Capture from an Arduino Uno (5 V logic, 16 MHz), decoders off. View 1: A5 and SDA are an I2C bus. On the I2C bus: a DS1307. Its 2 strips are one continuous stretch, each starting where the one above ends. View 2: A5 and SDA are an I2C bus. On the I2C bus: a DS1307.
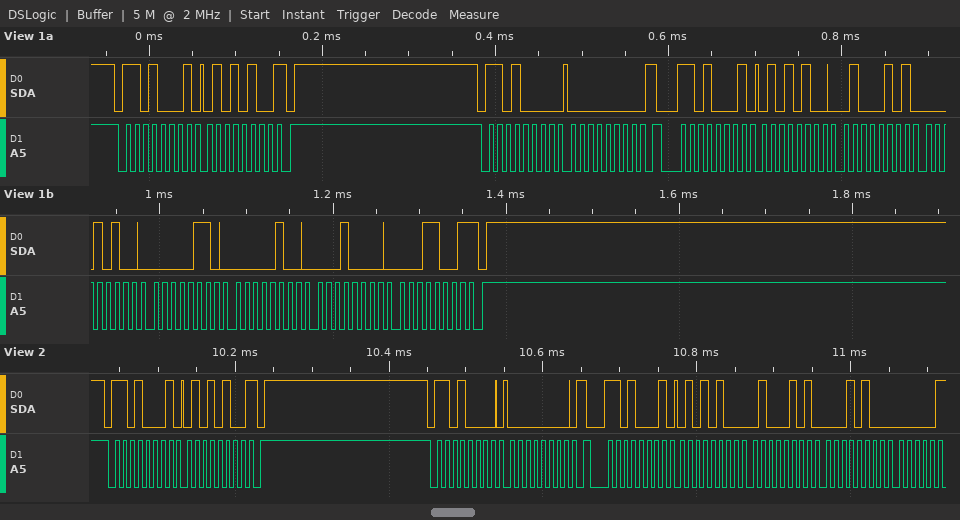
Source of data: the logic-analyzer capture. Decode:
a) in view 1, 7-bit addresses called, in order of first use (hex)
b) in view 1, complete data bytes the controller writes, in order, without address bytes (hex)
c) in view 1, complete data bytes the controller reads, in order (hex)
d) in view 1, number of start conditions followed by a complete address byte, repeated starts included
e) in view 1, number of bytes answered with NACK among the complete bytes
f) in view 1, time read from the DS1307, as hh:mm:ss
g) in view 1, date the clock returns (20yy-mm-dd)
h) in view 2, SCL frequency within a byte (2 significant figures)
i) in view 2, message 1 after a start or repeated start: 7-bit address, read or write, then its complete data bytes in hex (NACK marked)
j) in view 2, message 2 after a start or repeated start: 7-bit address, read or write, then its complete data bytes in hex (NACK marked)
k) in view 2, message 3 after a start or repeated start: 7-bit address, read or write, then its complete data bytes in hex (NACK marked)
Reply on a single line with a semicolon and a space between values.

0x68; 00; 54 54 45 14 06 04 10 19; 3; 2; 14:45:54; 2019-10-04; 100 kHz; 0x68 read: 54 NACK; 0x68 write: 00; 0x68 read: 54 45 14
